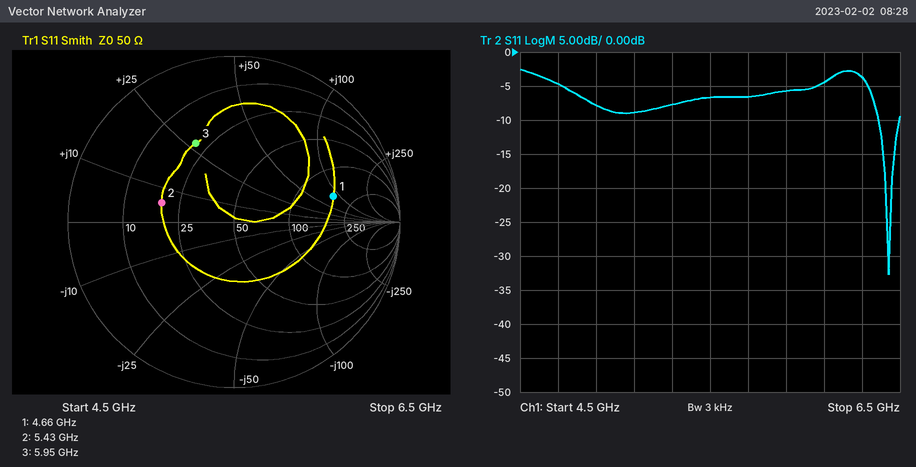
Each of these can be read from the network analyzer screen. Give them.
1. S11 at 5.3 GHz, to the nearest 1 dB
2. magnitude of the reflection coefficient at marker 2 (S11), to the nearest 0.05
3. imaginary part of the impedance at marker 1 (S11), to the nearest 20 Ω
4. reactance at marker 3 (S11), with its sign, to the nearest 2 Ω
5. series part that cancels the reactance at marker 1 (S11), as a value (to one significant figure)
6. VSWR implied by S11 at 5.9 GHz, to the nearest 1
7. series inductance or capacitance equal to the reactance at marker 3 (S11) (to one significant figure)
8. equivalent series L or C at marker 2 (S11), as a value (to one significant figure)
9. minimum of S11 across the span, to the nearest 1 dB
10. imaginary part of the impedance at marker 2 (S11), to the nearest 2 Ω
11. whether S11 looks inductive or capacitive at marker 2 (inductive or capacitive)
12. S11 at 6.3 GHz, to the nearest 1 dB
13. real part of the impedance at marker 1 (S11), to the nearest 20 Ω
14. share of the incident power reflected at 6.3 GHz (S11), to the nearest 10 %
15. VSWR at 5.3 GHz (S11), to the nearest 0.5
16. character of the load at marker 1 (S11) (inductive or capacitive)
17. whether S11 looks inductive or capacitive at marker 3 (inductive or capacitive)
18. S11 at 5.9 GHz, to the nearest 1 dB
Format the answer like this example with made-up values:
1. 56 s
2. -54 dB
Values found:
1. -8 dB
2. 0.45
3. +80 Ω
4. +28 Ω
5. 400 fF
6. 3
7. 700 pH
8. 200 pH
9. -33 dB
10. +6 Ω
11. inductive
12. -4 dB
13. 160 Ω
14. 40 %
15. 2.5
16. inductive
17. inductive
18. -6 dB
